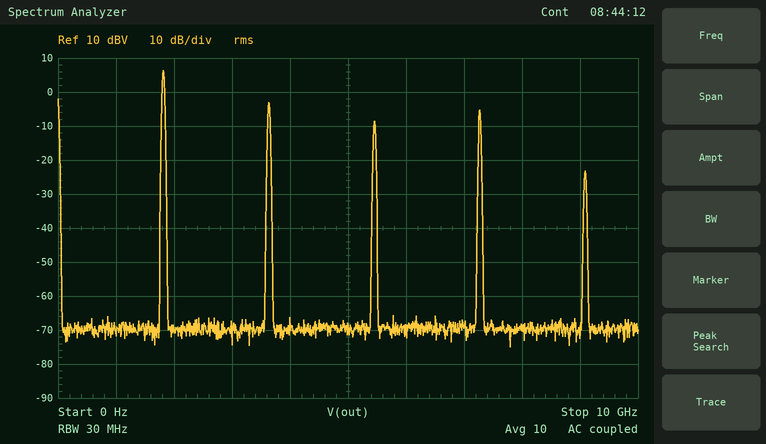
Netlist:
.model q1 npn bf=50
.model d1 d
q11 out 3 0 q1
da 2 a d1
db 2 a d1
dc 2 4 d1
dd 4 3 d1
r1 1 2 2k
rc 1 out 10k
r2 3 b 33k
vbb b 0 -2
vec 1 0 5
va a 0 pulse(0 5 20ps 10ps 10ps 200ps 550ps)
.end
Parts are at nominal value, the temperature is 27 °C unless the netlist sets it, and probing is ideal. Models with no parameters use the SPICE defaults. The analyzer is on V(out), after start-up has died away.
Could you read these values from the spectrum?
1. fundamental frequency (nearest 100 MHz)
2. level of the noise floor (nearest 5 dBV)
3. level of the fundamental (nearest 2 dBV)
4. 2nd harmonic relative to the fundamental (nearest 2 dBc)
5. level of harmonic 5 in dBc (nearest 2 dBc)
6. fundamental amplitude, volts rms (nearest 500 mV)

1.8 GHz
-70 dBV
6 dBV
-10 dBc
-30 dBc
2.0 V
